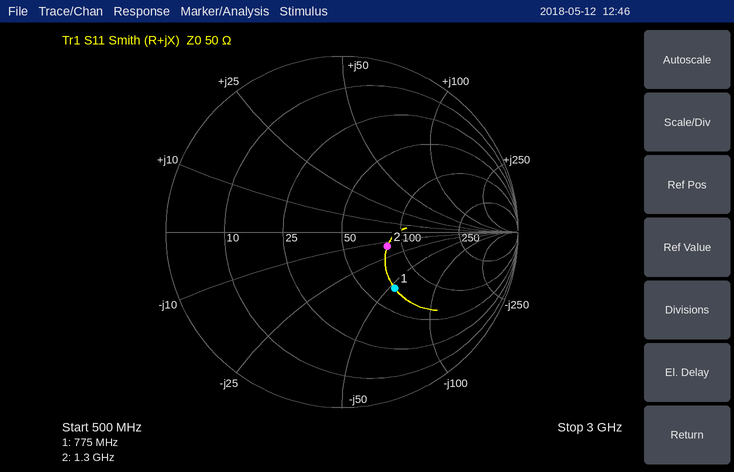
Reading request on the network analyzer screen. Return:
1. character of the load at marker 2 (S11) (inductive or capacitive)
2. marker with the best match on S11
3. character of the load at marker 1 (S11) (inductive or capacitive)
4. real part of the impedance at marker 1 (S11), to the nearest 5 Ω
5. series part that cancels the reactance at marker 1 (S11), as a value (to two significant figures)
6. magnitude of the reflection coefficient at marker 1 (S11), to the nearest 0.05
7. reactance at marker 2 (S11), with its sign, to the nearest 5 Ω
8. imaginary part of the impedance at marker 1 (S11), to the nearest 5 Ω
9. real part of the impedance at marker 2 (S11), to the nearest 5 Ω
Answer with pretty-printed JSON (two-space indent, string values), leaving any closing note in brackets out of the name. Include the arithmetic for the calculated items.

{
  "character of the load at marker 2 (S11)": "capacitive",
  "marker with the best match on S11": "marker 2",
  "character of the load at marker 1 (S11)": "capacitive",
  "real part of the impedance at marker 1 (S11), to the nearest 5 Ω": "70 Ω",
  "series part that cancels the reactance at marker 1 (S11), as a value": "L = 55 Ω/(2π × 775 MHz) ≈ 11 nH",
  "magnitude of the reflection coefficient at marker 1 (S11), to the nearest 0.05": "0.45",
  "reactance at marker 2 (S11), with its sign, to the nearest 5 Ω": "-15 Ω",
  "imaginary part of the impedance at marker 1 (S11), to the nearest 5 Ω": "-55 Ω",
  "real part of the impedance at marker 2 (S11), to the nearest 5 Ω": "85 Ω"
}
